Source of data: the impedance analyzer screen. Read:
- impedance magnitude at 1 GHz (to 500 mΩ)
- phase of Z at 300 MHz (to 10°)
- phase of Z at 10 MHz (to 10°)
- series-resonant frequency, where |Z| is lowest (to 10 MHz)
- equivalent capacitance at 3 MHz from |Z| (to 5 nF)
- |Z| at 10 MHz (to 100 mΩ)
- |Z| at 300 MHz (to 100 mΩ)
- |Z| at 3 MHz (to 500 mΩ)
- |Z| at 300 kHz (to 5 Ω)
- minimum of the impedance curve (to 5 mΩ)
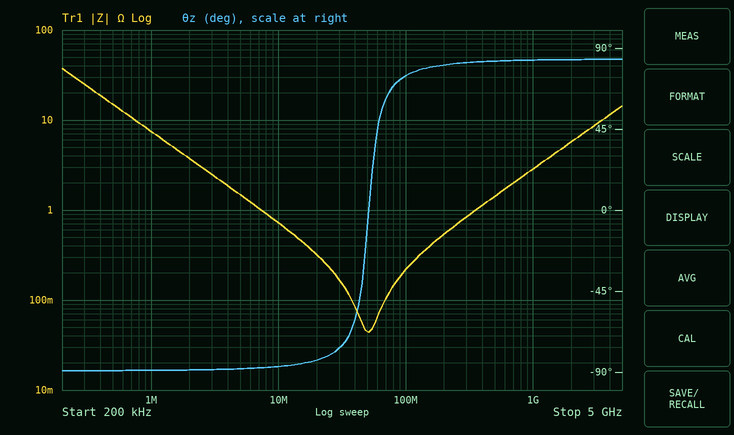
3.0 Ω
80°
-90°
50 MHz
20 nF
700 mΩ
800 mΩ
2.5 Ω
25 Ω
45 mΩ
